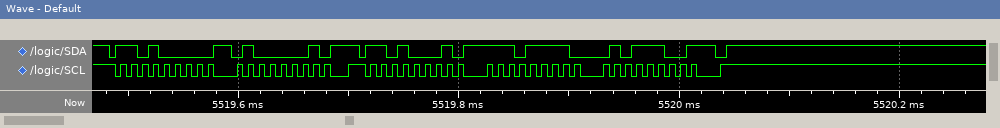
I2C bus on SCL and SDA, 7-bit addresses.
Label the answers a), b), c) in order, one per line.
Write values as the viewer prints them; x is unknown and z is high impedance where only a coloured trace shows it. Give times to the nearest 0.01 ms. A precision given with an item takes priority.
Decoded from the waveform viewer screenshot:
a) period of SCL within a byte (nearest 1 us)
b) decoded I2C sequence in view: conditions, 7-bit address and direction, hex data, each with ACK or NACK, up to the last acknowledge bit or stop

a) 10 us
b) start, address 68 write ACK, 41 ACK, repeated start, address 68 read ACK, EF ACK, 5C NACK, stop
